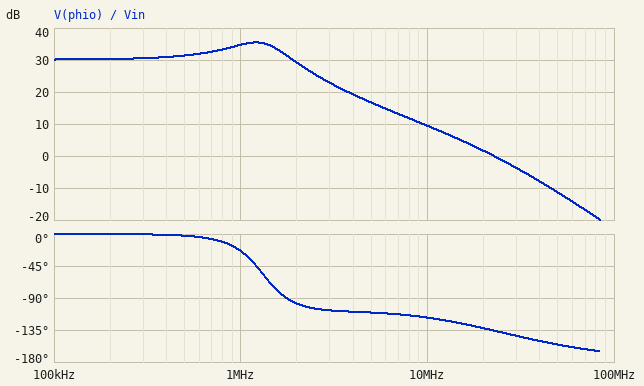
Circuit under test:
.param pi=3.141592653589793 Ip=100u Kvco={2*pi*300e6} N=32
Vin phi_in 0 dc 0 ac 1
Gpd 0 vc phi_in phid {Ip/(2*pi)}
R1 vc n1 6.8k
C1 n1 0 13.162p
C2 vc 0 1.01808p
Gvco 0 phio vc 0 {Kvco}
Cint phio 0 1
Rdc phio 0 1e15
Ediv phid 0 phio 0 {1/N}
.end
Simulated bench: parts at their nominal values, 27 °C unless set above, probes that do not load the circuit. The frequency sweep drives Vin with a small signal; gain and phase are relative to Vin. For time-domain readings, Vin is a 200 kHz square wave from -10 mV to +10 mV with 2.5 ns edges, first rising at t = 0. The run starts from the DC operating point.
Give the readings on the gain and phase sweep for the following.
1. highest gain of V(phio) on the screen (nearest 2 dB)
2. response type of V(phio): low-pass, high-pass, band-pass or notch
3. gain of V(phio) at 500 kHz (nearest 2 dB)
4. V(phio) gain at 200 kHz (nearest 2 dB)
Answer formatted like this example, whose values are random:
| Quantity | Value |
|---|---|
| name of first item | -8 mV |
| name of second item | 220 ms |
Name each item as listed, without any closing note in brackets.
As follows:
| Quantity | Value |
|---|---|
| highest gain of V(phio) on the screen | 36 dB |
| response type of V(phio): low-pass, high-pass, band-pass or notch | low-pass |
| gain of V(phio) at 500 kHz | 32 dB |
| V(phio) gain at 200 kHz | 30 dB |
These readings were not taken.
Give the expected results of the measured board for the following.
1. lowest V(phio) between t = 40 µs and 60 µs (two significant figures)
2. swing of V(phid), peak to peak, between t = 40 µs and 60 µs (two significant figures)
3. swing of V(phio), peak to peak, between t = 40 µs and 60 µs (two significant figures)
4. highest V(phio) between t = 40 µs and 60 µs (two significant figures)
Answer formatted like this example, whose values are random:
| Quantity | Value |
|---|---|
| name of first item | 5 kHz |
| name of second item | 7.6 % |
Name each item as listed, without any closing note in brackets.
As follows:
| Quantity | Value |
|---|---|
| lowest V(phio) between t = 40 µs and 60 µs | -590 mV |
| swing of V(phid), peak to peak, between t = 40 µs and 60 µs | 37 mV |
| swing of V(phio), peak to peak, between t = 40 µs and 60 µs | 1.2 V |
| highest V(phio) between t = 40 µs and 60 µs | 590 mV |
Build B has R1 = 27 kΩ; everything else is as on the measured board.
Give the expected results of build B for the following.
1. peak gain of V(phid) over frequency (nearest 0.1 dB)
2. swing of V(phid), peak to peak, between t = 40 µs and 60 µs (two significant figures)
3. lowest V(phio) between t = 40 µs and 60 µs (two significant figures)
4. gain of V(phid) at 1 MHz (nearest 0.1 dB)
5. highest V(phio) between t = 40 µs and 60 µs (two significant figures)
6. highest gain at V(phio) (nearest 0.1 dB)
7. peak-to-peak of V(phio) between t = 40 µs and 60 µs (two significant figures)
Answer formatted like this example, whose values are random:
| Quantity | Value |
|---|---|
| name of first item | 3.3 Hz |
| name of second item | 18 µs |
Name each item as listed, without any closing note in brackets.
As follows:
| Quantity | Value |
|---|---|
| peak gain of V(phid) over frequency | 1.3 dB |
| swing of V(phid), peak to peak, between t = 40 µs and 60 µs | 28 mV |
| lowest V(phio) between t = 40 µs and 60 µs | -450 mV |
| gain of V(phid) at 1 MHz | 1.0 dB |
| highest V(phio) between t = 40 µs and 60 µs | 450 mV |
| highest gain at V(phio) | 31.4 dB |
| peak-to-peak of V(phio) between t = 40 µs and 60 µs | 900 mV |
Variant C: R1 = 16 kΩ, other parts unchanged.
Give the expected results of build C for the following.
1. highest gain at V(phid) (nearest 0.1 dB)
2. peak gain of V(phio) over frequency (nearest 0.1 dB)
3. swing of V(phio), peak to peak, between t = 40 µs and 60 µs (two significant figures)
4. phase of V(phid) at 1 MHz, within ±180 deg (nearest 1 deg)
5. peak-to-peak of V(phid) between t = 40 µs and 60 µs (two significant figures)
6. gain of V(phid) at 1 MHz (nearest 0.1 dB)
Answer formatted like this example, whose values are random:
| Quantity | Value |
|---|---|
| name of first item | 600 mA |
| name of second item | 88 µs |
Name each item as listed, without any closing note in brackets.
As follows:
| Quantity | Value |
|---|---|
| highest gain at V(phid) | 2.0 dB |
| peak gain of V(phio) over frequency | 32.1 dB |
| swing of V(phio), peak to peak, between t = 40 µs and 60 µs | 910 mV |
| phase of V(phid) at 1 MHz, within ±180 deg | -19 deg |
| peak-to-peak of V(phid) between t = 40 µs and 60 µs | 28 mV |
| gain of V(phid) at 1 MHz | 1.9 dB |
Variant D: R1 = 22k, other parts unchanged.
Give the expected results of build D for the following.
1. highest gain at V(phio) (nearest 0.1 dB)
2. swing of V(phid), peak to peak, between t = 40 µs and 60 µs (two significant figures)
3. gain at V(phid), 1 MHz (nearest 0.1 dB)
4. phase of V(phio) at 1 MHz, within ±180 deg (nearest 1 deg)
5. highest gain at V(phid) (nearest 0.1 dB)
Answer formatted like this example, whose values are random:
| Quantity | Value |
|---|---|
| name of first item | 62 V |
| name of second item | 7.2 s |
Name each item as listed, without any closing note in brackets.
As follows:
| Quantity | Value |
|---|---|
| highest gain at V(phio) | 31.5 dB |
| swing of V(phid), peak to peak, between t = 40 µs and 60 µs | 27 mV |
| gain at V(phid), 1 MHz | 1.3 dB |
| phase of V(phio) at 1 MHz, within ±180 deg | -16 deg |
| highest gain at V(phid) | 1.4 dB |
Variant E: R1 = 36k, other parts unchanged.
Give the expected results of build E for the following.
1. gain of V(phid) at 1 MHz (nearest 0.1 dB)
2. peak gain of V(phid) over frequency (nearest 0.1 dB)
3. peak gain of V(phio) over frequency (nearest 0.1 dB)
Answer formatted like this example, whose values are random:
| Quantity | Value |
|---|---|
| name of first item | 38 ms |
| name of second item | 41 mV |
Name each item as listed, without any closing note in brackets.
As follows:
| Quantity | Value |
|---|---|
| gain of V(phid) at 1 MHz | 0.8 dB |
| peak gain of V(phid) over frequency | 2.3 dB |
| peak gain of V(phio) over frequency | 32.4 dB |
